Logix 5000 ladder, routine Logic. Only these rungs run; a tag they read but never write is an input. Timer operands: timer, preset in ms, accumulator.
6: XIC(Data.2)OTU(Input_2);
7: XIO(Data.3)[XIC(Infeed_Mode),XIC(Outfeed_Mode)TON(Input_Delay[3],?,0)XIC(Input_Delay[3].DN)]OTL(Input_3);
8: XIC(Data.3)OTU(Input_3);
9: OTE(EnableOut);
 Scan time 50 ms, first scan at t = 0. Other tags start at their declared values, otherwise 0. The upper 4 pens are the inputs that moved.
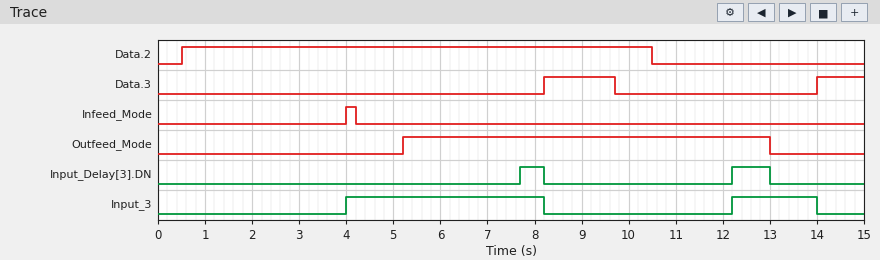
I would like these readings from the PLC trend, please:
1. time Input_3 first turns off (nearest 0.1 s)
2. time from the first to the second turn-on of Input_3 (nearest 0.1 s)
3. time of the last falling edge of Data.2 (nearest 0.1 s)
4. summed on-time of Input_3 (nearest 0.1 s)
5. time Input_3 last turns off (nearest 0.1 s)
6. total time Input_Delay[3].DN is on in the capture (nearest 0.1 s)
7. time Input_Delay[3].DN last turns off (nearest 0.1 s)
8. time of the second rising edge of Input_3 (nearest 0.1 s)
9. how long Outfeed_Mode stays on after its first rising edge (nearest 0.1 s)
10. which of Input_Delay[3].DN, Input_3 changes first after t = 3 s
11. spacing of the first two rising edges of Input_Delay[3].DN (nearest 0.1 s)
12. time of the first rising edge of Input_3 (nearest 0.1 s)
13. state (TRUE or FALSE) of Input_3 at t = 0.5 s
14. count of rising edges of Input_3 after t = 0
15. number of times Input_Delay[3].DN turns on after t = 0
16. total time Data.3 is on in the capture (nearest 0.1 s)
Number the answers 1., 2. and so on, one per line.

1. 8.2 s
2. 8.2 s
3. 10.5 s
4. 6.0 s
5. 14.0 s
6. 1.3 s
7. 13.0 s
8. 12.2 s
9. 7.8 s
10. Input_3
11. 4.5 s
12. 4.0 s
13. FALSE
14. 2
15. 2
16. 2.5 s
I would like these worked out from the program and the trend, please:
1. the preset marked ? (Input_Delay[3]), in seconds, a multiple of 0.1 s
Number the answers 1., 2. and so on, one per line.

1. 2.5 s
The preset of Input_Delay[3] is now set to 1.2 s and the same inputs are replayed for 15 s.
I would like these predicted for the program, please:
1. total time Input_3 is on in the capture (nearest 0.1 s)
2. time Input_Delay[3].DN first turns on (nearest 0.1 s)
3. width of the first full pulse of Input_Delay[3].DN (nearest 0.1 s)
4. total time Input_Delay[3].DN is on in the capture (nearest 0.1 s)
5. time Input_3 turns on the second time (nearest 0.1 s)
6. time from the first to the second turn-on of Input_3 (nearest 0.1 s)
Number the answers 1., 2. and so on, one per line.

1. 7.3 s
2. 6.4 s
3. 1.8 s
4. 3.9 s
5. 10.9 s
6. 6.9 s
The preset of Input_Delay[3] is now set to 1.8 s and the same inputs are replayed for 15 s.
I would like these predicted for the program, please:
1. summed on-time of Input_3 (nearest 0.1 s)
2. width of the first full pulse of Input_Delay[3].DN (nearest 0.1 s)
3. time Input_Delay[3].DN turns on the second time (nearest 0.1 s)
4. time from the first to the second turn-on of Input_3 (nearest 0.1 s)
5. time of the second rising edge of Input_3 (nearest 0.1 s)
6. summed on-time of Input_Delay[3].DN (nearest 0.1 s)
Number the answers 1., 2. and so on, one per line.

1. 6.7 s
2. 1.2 s
3. 11.5 s
4. 7.5 s
5. 11.5 s
6. 2.7 s
